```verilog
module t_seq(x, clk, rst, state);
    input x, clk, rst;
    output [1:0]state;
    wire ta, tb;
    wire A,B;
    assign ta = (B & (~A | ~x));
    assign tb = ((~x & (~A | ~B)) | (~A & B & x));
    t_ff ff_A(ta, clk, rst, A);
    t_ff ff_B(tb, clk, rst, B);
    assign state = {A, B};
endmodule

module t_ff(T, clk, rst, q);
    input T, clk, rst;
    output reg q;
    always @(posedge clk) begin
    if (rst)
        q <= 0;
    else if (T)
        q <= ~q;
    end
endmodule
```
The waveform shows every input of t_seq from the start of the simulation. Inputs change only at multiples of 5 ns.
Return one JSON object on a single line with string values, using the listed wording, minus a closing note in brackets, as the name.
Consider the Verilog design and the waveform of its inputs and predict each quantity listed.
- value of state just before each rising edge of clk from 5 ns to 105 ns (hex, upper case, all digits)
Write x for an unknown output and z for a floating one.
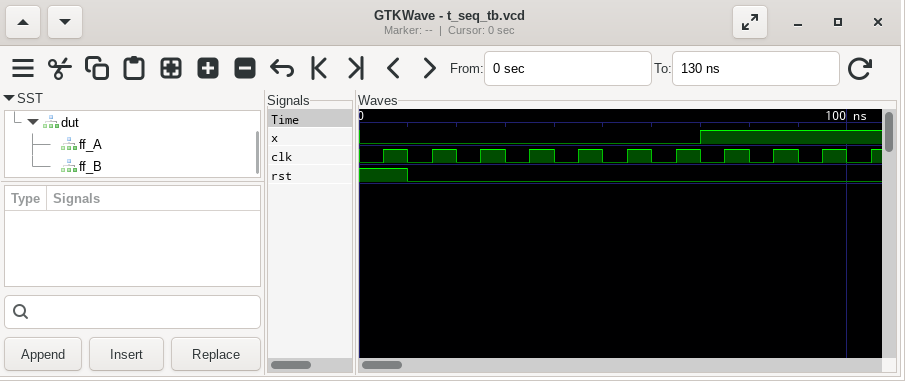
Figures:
{"value of state just before each rising edge of clk from 5 ns to 105 ns": "x, 0, 1, 2, 3, 1, 2, 3, 3, 3, 3"}
